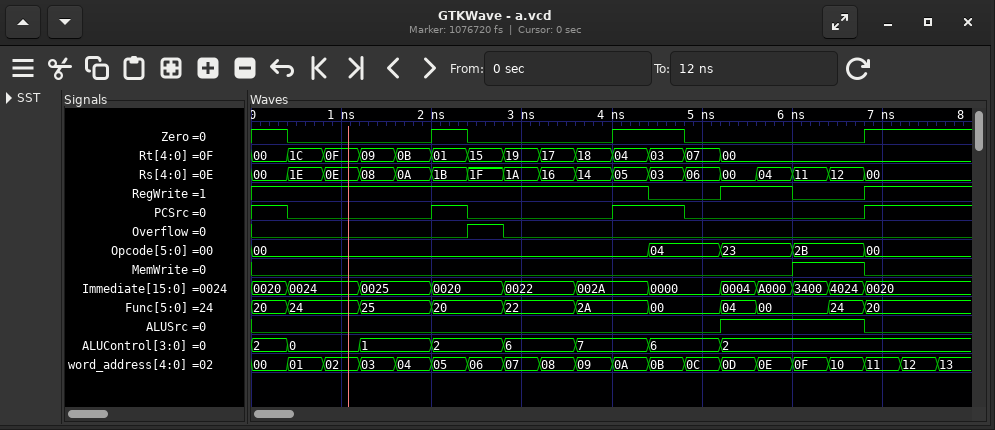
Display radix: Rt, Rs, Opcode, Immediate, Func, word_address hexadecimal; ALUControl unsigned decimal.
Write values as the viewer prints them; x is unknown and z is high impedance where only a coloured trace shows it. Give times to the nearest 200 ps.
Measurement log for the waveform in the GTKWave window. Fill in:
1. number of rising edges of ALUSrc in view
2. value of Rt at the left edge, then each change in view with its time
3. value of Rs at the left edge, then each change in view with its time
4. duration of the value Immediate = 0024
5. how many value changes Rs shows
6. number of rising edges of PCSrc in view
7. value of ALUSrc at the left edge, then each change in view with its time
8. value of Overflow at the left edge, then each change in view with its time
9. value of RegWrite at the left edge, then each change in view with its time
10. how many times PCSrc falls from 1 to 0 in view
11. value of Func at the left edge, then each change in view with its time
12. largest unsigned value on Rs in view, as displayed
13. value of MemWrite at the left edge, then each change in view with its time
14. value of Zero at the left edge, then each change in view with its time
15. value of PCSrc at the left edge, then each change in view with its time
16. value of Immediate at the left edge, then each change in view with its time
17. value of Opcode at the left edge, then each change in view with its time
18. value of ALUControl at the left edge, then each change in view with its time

1
00, 1C at 400 ps, 0F at 800 ps, 09 at 1200 ps, 0B at 1600 ps, 01 at 2000 ps, 15 at 2400 ps, 19 at 2800 ps, 17 at 3200 ps, 18 at 3600 ps, 04 at 4000 ps, 03 at 4400 ps, 07 at 4800 ps, 00 at 5200 ps
00, 1E at 400 ps, 0E at 800 ps, 08 at 1200 ps, 0A at 1600 ps, 1B at 2000 ps, 1F at 2400 ps, 1A at 2800 ps, 16 at 3200 ps, 14 at 3600 ps, 05 at 4000 ps, 03 at 4400 ps, 06 at 4800 ps, 00 at 5200 ps, 04 at 5600 ps, 11 at 6000 ps, 12 at 6400 ps, 00 at 6800 ps
800 ps
17
3
0, 1 at 5200 ps, 0 at 6800 ps
0, 1 at 2400 ps, 0 at 2800 ps
1, 0 at 4400 ps, 1 at 5200 ps, 0 at 6000 ps, 1 at 6800 ps
3
20, 24 at 400 ps, 25 at 1200 ps, 20 at 2000 ps, 22 at 2800 ps, 2A at 3600 ps, 00 at 4400 ps, 04 at 5200 ps, 00 at 5600 ps, 24 at 6400 ps, 20 at 6800 ps
1F
0, 1 at 6000 ps, 0 at 6800 ps
1, 0 at 400 ps, 1 at 2000 ps, 0 at 2400 ps, 1 at 4000 ps, 0 at 4800 ps, 1 at 6800 ps
1, 0 at 400 ps, 1 at 2000 ps, 0 at 2400 ps, 1 at 4000 ps, 0 at 4800 ps, 1 at 6800 ps
0020, 0024 at 400 ps, 0025 at 1200 ps, 0020 at 2000 ps, 0022 at 2800 ps, 002A at 3600 ps, 0000 at 4400 ps, 0004 at 5200 ps, A000 at 5600 ps, 3400 at 6000 ps, 4024 at 6400 ps, 0020 at 6800 ps
00, 04 at 4400 ps, 23 at 5200 ps, 2B at 6000 ps, 00 at 6800 ps
2, 0 at 400 ps, 1 at 1200 ps, 2 at 2000 ps, 6 at 2800 ps, 7 at 3600 ps, 6 at 4400 ps, 2 at 5200 ps
